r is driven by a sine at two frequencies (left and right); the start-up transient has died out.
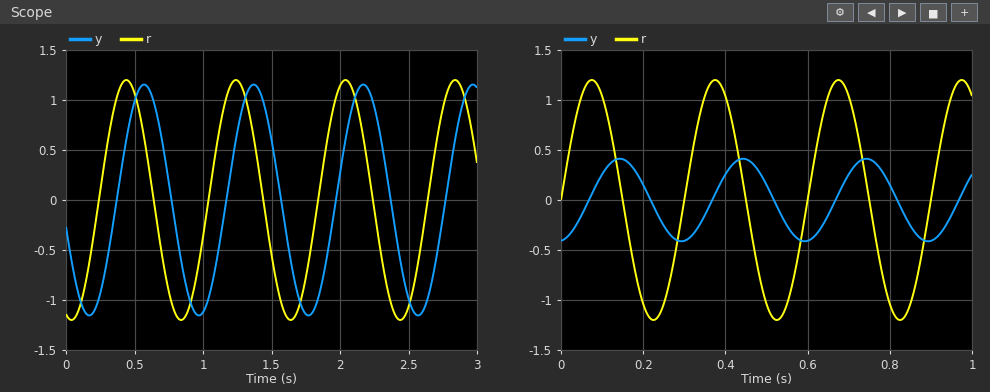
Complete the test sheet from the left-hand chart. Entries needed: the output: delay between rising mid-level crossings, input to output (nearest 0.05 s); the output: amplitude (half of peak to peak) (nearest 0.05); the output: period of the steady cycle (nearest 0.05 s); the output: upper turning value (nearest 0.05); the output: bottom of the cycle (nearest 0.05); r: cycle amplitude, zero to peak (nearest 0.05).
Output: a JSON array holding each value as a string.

["0.15 s", "1.15", "0.80 s", "1.15", "-1.15", "1.20"]
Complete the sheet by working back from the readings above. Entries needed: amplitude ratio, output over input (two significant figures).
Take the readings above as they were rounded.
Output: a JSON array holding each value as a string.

["0.96"]
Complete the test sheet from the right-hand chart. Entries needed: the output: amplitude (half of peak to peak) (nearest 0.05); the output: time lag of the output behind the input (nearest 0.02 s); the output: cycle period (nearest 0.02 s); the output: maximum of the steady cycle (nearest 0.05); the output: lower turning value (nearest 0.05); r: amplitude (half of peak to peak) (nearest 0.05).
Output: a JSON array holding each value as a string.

["0.40", "0.06 s", "0.30 s", "0.40", "-0.40", "1.20"]
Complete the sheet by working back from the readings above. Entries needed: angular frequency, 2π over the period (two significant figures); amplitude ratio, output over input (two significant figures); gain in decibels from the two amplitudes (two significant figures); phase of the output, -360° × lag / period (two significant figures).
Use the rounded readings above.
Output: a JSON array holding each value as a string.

["21 rad/s", "0.33", "-9.5 dB", "-72°"]
